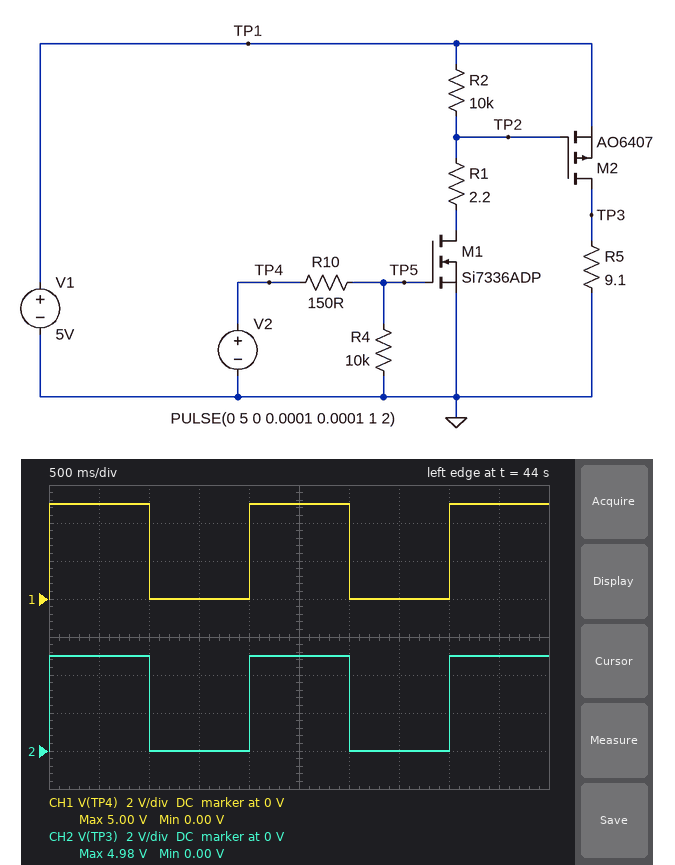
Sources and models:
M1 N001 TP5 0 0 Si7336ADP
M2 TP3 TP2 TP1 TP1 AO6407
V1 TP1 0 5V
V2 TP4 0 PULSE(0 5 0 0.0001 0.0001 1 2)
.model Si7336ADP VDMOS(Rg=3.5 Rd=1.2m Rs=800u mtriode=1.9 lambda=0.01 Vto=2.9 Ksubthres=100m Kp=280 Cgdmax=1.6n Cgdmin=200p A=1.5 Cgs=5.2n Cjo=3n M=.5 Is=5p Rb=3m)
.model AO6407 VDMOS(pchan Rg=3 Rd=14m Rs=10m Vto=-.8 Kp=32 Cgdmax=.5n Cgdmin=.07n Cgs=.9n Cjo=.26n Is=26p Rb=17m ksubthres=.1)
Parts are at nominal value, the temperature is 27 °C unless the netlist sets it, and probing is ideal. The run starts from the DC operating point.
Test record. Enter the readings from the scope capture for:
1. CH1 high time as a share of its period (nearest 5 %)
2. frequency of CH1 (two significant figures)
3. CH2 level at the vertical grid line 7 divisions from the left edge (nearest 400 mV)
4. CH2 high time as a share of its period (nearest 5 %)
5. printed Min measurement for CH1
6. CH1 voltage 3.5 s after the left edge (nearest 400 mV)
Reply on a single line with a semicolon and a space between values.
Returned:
50 %; 500 mHz; 0 V; 50 %; 0.00 V; 0 V
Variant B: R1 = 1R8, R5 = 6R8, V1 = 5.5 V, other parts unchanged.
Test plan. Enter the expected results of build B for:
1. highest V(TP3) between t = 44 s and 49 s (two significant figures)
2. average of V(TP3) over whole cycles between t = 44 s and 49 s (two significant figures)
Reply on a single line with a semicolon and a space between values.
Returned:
5.5 V; 2.7 V
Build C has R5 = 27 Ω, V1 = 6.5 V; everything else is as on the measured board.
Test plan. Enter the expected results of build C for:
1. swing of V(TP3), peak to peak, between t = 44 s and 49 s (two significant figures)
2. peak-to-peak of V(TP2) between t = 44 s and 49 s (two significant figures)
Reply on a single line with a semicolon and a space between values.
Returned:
6.5 V; 6.6 V
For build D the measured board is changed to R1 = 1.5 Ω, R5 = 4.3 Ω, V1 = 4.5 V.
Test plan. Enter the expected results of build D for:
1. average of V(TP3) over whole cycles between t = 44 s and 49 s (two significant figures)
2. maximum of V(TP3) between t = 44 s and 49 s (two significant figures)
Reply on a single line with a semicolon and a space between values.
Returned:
2.2 V; 4.5 V
